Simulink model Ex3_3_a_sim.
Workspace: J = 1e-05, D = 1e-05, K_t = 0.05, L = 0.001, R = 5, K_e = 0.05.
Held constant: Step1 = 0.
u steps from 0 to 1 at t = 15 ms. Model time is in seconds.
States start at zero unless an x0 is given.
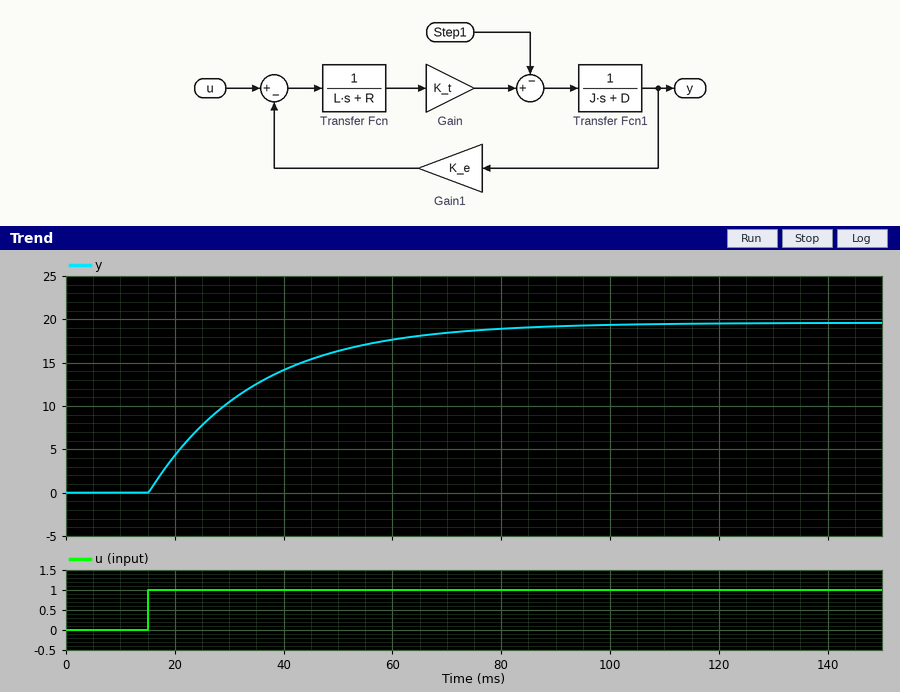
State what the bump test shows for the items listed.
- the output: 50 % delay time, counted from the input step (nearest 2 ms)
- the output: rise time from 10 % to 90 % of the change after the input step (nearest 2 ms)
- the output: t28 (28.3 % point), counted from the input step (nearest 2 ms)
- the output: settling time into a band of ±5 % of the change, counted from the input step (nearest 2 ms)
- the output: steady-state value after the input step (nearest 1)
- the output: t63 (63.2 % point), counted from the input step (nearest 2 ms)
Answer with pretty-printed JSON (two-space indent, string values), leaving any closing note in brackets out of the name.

{
  "the output: 50 % delay time, counted from the input step": "14 ms",
  "the output: rise time from 10 % to 90 % of the change after the input step": "42 ms",
  "the output: t28 (28.3 % point), counted from the input step": "6 ms",
  "the output: settling time into a band of ±5 % of the change, counted from the input step": "58 ms",
  "the output: steady-state value after the input step": "20",
  "the output: t63 (63.2 % point), counted from the input step": "20 ms"
}
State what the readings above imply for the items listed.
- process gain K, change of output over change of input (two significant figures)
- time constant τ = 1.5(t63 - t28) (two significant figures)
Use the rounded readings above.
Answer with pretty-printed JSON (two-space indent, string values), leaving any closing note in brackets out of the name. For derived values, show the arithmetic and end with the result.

{
  "process gain K, change of output over change of input": "(20 - 0) / 1 = 20",
  "time constant τ = 1.5(t63 - t28)": "1.5 × (20 - 6) = 21 ms"
}
